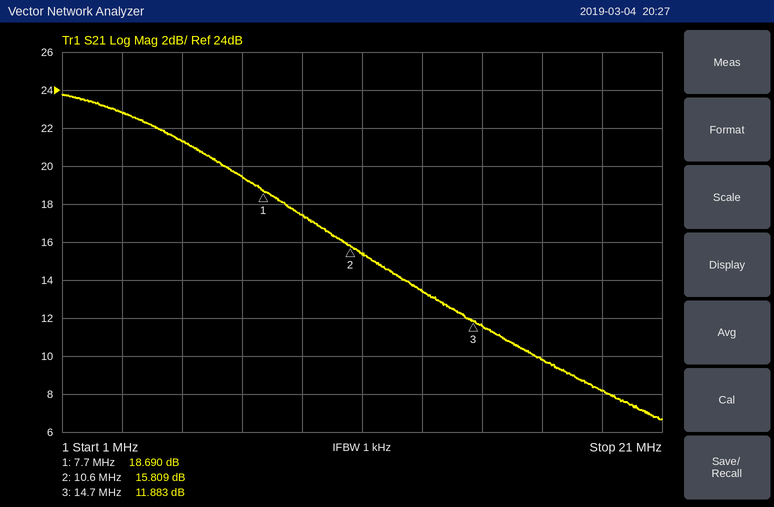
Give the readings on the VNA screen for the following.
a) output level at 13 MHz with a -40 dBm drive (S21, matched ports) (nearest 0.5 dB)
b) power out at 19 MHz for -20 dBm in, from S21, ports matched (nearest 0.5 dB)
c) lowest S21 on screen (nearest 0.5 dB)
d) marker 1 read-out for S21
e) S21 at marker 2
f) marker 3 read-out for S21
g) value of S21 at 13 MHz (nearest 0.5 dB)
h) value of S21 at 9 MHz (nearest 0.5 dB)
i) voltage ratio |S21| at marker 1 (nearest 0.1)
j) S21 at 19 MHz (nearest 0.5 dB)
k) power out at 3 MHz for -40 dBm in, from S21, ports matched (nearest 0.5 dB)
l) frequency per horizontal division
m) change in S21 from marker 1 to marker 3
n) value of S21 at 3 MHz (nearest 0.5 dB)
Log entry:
-26.5 dBm
-12.0 dBm
6.5 dB
18.690 dB
15.809 dB
11.883 dB
13.5 dB
17.5 dB
8.6
8.0 dB
-17.0 dBm
2 MHz
-6.807 dB
23.0 dB
